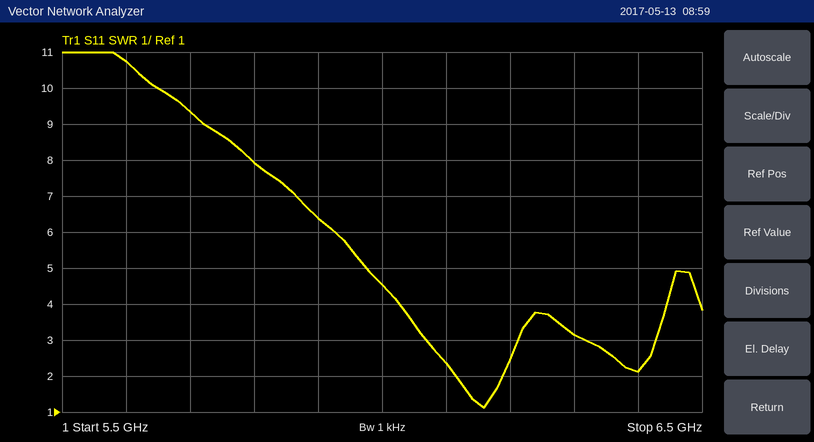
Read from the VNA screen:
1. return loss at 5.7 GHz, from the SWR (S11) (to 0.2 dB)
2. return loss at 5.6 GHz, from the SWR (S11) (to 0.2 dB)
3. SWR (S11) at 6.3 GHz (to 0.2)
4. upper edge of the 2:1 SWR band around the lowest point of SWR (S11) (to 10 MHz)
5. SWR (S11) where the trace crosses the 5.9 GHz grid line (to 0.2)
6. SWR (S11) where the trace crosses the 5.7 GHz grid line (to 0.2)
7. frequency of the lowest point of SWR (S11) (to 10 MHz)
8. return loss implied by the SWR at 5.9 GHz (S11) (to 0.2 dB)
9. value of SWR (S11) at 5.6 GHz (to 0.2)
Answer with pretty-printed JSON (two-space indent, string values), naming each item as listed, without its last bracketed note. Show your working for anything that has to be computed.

{
  "return loss at 5.7 GHz, from the SWR (S11)": "−20 log10((9.4 − 1)/(9.4 + 1)) ≈ 1.86 dB, so 1.8 dB to the nearest 0.2 dB",
  "return loss at 5.6 GHz, from the SWR (S11)": "−20 log10((10.8 − 1)/(10.8 + 1)) ≈ 1.6 dB",
  "SWR (S11) at 6.3 GHz": "3.2",
  "upper edge of the 2:1 SWR band around the lowest point of SWR (S11)": "6.19 GHz",
  "SWR (S11) where the trace crosses the 5.9 GHz grid line": "6.4",
  "SWR (S11) where the trace crosses the 5.7 GHz grid line": "9.4",
  "frequency of the lowest point of SWR (S11)": "6.16 GHz",
  "return loss implied by the SWR at 5.9 GHz (S11)": "−20 log10((6.4 − 1)/(6.4 + 1)) ≈ 2.74 dB, so 2.8 dB to the nearest 0.2 dB",
  "value of SWR (S11) at 5.6 GHz": "10.8"
}
